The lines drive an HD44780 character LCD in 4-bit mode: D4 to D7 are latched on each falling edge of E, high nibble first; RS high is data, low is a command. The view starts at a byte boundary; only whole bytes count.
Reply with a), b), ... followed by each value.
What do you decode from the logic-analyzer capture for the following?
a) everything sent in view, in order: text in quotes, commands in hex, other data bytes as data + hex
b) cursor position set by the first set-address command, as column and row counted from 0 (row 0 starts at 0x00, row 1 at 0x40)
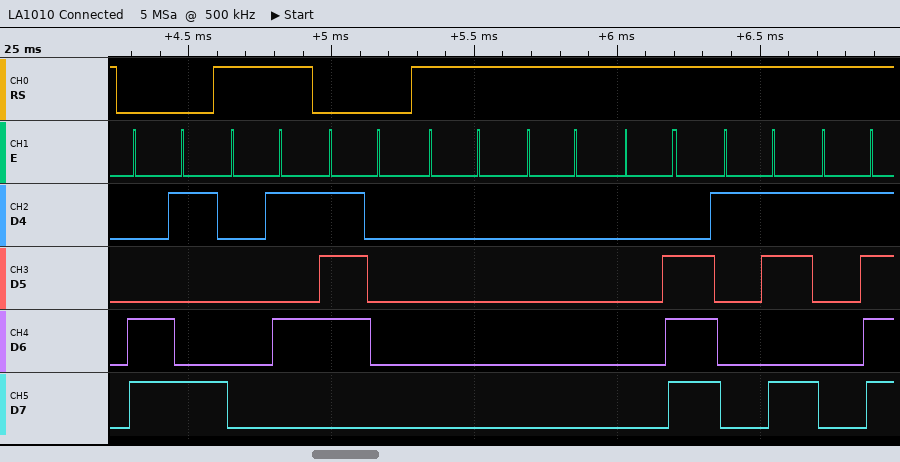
a) 0xC9 data 05 0x70 data 00 00 0E 1B 1F
b) column 9, row 1
